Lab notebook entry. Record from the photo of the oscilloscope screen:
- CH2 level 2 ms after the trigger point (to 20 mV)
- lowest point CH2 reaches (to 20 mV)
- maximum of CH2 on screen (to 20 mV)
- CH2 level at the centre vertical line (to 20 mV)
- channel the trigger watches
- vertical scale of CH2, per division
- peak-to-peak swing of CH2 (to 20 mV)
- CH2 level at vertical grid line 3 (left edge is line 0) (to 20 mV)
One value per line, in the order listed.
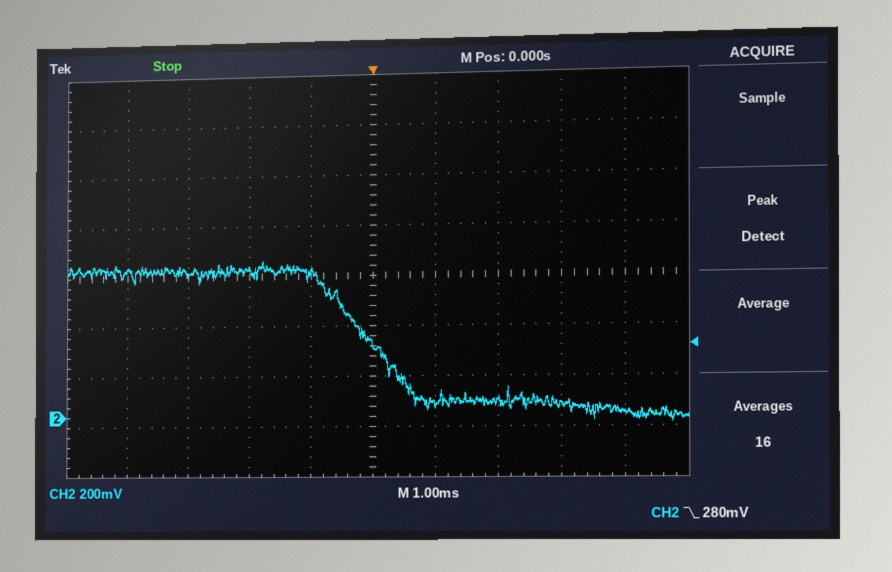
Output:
60 mV
-20 mV
620 mV
280 mV
CH2
200 mV
640 mV
580 mV
